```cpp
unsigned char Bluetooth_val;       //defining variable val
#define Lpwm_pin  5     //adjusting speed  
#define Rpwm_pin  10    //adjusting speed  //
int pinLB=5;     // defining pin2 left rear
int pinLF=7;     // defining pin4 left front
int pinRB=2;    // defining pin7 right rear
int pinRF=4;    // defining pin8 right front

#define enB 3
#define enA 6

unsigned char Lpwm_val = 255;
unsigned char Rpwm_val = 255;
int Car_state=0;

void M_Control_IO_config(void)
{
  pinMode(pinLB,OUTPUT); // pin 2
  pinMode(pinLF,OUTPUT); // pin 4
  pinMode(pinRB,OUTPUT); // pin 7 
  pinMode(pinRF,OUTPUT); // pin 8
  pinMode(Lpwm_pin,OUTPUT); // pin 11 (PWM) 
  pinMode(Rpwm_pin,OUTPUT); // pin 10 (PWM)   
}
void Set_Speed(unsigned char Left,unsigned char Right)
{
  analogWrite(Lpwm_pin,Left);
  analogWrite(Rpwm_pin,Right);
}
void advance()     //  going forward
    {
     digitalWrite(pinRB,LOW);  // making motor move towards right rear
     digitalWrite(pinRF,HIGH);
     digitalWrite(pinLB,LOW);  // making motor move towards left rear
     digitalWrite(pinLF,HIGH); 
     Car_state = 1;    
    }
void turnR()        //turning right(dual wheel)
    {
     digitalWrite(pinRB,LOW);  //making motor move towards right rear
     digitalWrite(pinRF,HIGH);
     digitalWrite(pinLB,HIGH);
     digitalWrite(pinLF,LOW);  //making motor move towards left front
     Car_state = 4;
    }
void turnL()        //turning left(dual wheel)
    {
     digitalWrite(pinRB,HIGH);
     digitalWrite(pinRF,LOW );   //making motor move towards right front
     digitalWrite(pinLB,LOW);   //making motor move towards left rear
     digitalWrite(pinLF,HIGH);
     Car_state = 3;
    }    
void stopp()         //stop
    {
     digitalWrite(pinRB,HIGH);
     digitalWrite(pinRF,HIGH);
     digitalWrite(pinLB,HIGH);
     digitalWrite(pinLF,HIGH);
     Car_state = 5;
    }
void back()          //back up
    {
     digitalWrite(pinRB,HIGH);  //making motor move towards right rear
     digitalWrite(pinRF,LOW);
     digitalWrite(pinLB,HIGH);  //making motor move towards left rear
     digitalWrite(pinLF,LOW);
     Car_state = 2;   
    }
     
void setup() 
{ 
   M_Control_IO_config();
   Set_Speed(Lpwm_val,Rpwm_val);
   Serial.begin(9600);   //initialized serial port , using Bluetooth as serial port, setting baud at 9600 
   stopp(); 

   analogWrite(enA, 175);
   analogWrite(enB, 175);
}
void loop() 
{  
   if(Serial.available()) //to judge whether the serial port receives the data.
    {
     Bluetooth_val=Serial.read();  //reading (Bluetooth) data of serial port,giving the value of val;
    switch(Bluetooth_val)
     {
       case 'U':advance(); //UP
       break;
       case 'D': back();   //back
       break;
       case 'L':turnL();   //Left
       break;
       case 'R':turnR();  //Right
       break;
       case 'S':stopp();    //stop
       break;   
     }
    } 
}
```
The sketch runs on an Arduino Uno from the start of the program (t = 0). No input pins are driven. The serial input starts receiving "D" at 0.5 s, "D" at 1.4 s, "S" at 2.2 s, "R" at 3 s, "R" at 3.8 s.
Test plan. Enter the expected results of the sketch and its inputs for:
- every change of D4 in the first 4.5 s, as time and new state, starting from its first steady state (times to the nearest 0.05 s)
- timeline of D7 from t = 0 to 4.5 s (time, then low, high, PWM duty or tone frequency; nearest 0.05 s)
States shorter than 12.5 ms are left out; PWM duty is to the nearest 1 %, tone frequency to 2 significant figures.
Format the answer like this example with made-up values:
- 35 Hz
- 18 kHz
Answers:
- 0 s high; 0.5 s low; 2.2 s high
- 0 s high; 0.5 s low; 2.2 s high; 3 s low
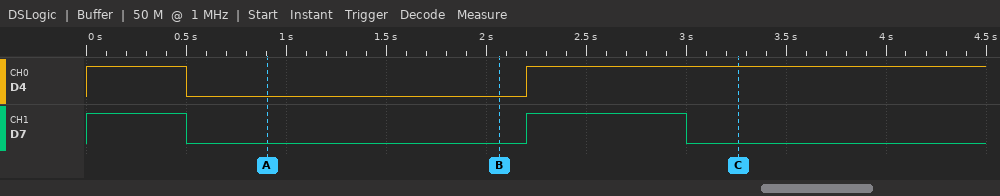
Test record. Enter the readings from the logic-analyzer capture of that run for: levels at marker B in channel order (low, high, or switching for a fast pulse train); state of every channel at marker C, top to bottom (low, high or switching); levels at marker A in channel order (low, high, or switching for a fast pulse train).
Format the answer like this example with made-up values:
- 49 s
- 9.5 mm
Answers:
- D4 low, D7 low
- D4 high, D7 low
- D4 low, D7 low
